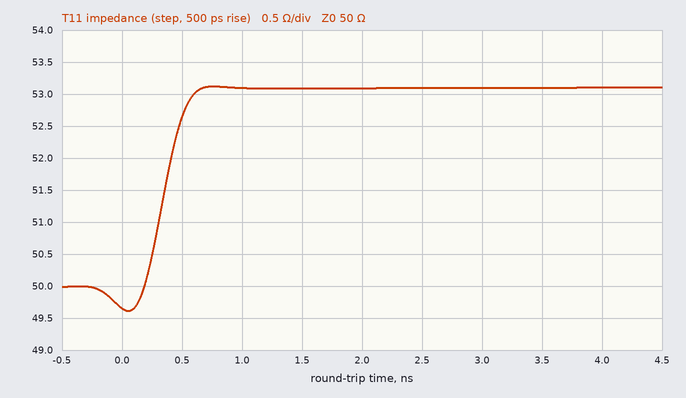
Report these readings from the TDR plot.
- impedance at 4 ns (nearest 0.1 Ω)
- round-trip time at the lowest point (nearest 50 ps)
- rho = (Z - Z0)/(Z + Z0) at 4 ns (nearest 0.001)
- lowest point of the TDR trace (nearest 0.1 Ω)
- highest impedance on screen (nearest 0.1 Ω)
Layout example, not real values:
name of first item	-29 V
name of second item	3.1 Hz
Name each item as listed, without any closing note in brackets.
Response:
impedance at 4 ns	53.1 Ω
round-trip time at the lowest point	50 ps
rho = (Z - Z0)/(Z + Z0) at 4 ns	+0.030
lowest point of the TDR trace	49.6 Ω
highest impedance on screen	53.1 Ω
